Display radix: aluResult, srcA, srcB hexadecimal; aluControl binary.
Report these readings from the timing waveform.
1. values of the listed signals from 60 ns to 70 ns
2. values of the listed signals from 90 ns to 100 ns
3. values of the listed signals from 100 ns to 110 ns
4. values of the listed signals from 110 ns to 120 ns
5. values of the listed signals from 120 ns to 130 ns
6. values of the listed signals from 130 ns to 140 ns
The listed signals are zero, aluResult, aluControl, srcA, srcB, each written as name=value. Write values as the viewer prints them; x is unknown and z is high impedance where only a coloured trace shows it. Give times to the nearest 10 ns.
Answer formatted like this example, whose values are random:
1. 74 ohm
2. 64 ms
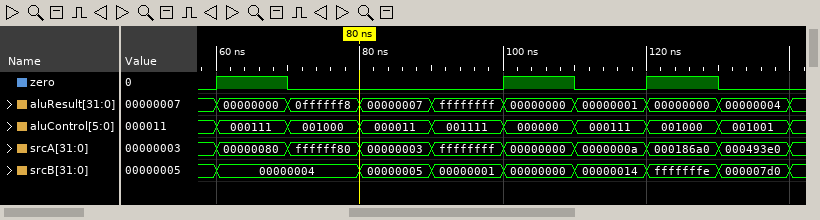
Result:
1. zero=1, aluResult=00000000, aluControl=000111, srcA=00000080, srcB=00000004
2. zero=0, aluResult=ffffffff, aluControl=001111, srcA=ffffffff, srcB=00000001
3. zero=1, aluResult=00000000, aluControl=000000, srcA=00000000, srcB=00000000
4. zero=0, aluResult=00000001, aluControl=000111, srcA=0000000a, srcB=00000014
5. zero=1, aluResult=00000000, aluControl=001000, srcA=000186a0, srcB=fffffffe
6. zero=0, aluResult=00000004, aluControl=001001, srcA=000493e0, srcB=000007d0
